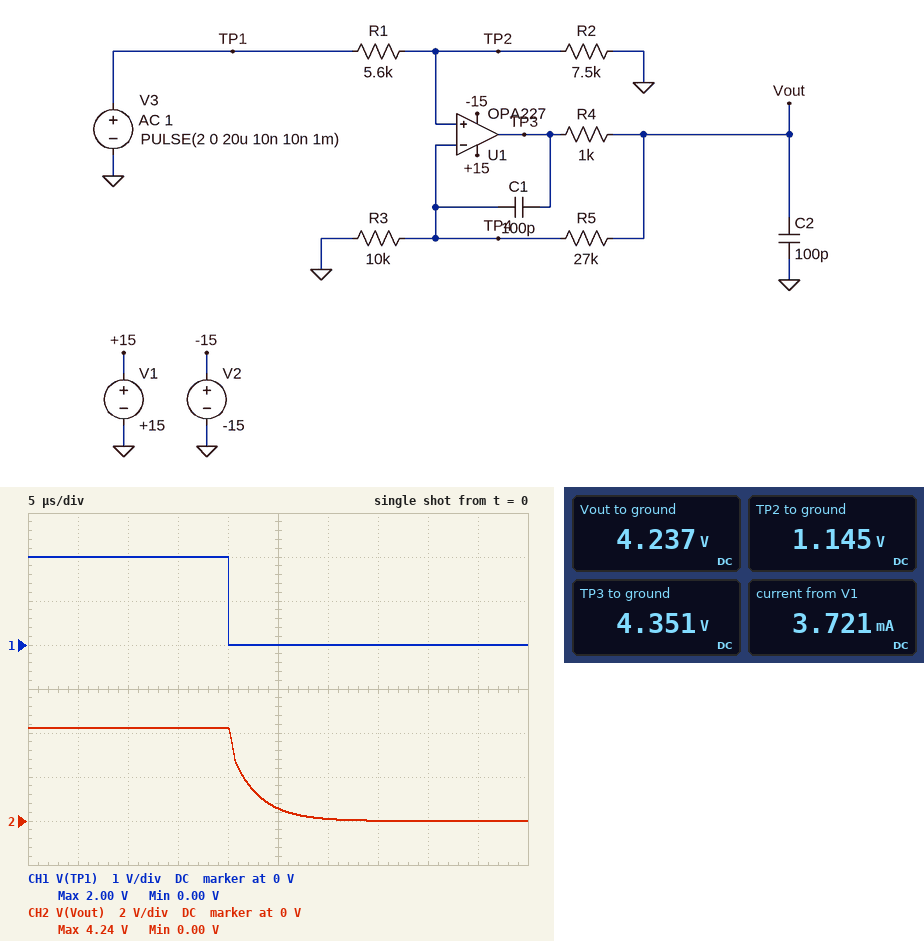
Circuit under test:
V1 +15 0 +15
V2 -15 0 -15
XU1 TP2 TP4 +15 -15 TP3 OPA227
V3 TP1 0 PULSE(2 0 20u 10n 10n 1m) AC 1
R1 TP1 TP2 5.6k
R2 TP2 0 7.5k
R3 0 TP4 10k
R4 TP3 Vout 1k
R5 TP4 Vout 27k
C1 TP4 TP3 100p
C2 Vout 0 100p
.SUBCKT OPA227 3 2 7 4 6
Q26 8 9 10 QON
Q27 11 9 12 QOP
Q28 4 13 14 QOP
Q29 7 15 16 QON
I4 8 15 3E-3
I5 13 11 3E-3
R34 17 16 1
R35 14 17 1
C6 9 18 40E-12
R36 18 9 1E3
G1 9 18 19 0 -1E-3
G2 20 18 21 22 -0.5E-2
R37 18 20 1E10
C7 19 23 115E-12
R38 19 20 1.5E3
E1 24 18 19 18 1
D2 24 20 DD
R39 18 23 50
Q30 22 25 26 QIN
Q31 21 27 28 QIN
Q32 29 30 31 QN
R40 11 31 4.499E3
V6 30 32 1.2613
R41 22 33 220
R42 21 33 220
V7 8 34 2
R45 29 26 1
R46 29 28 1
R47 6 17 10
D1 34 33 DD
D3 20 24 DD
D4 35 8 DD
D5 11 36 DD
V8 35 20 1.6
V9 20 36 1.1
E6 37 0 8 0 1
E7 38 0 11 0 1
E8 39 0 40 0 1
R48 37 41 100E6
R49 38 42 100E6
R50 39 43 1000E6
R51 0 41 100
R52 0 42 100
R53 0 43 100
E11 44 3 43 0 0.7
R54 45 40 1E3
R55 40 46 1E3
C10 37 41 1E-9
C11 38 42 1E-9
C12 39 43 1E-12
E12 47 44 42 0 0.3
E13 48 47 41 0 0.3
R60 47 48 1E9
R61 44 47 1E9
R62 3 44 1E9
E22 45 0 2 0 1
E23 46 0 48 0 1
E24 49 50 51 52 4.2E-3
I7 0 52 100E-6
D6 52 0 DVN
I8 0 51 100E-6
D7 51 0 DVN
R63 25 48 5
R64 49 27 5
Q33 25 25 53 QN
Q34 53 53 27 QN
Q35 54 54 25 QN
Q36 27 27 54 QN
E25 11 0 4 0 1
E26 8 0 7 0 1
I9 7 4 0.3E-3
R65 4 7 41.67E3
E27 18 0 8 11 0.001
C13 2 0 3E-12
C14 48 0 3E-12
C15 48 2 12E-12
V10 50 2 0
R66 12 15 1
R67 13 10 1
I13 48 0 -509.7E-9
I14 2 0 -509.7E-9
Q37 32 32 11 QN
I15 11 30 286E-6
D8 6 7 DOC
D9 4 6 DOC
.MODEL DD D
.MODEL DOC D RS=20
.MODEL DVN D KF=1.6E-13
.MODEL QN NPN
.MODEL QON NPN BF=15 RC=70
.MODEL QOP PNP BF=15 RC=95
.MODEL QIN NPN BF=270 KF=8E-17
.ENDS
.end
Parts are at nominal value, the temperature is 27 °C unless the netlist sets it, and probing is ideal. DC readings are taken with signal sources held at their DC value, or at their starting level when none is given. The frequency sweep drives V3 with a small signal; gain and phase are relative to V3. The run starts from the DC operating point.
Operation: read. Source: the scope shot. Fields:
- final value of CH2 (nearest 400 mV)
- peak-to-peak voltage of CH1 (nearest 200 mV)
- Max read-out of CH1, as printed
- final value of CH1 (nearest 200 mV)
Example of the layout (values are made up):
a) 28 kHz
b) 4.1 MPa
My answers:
a) 0 V
b) 2.0 V
c) 2.00 V
d) 0 V
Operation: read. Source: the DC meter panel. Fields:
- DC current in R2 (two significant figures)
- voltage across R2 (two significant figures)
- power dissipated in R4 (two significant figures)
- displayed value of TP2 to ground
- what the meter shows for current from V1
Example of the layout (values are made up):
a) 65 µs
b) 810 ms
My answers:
a) 150 µA
b) 1.1 V
c) 13 µW
d) 1.145 V
e) 3.721 mA
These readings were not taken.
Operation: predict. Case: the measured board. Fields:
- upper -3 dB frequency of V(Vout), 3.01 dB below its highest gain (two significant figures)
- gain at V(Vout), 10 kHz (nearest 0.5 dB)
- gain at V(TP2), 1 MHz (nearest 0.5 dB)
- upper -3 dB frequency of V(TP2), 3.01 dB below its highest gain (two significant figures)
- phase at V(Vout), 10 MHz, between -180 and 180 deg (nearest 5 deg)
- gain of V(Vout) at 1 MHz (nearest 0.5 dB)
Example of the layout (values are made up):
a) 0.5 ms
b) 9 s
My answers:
a) 63 kHz
b) 6.5 dB
c) -4.5 dB
d) 4.5 MHz
e) 70 deg
f) -5.5 dB
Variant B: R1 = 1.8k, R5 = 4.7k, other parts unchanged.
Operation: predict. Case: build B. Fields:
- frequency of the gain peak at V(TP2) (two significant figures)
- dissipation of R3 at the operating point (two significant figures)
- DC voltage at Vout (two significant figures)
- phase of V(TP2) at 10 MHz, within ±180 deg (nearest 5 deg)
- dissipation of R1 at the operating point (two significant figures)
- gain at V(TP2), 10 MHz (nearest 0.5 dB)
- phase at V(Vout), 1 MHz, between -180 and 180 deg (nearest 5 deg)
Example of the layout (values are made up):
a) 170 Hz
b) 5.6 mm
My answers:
a) 4.4 MHz
b) 260 µW
c) 2.4 V
d) -60 deg
e) 83 µW
f) -6.0 dB
g) -45 deg
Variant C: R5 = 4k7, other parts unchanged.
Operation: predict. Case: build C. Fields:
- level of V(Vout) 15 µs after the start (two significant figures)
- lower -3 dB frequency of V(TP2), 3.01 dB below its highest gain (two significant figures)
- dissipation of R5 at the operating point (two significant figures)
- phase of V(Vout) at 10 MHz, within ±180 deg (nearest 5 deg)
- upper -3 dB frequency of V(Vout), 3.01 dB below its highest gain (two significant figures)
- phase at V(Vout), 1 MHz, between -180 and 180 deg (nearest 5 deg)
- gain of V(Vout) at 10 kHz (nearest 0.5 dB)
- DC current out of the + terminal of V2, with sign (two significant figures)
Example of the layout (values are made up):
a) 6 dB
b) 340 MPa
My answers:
a) 1.7 V
b) 2.3 MHz
c) 62 µW
d) 75 deg
e) 1.3 MHz
f) -50 deg
g) -1.5 dB
h) -3.6 mA
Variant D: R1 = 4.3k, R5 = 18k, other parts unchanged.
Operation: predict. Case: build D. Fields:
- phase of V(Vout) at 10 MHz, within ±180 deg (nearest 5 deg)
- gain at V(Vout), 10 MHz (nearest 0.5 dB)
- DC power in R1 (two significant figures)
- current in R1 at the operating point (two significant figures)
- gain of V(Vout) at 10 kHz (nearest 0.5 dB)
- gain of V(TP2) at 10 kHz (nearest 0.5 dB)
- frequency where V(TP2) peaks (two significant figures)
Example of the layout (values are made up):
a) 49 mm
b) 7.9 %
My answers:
a) 75 deg
b) -38.0 dB
c) 120 µW
d) 170 µA
e) 5.0 dB
f) -4.0 dB
g) 3.9 MHz
